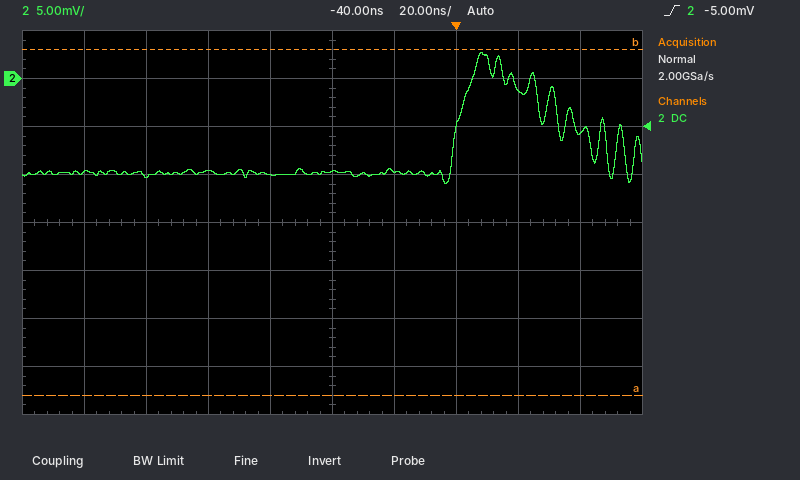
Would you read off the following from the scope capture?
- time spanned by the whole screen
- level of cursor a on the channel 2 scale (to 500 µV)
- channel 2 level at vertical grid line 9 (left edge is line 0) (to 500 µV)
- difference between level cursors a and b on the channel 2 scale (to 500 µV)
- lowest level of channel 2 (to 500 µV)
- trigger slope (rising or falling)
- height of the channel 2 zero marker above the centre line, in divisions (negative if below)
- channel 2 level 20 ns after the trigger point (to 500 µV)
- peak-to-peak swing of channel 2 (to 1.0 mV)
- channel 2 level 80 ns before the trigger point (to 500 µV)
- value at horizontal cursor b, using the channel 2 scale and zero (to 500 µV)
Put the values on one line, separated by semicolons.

200 ns; -33.0 mV; -5.5 mV; 36.0 mV; -11.0 mV; rising; +3.0 div; -1.0 mV; 14.0 mV; -9.5 mV; 3.0 mV
